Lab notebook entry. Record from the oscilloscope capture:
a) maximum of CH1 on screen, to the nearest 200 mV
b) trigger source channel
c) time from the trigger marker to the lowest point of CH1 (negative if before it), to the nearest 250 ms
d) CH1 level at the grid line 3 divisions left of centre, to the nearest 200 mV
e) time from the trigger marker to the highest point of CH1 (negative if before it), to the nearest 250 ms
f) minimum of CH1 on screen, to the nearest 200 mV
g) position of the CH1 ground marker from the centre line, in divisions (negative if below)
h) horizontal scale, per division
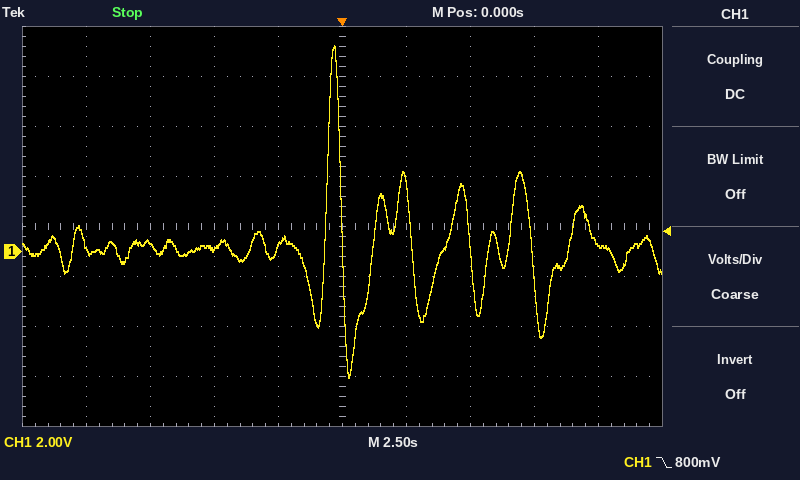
8.2 V
CH1
+250 ms
400 mV
-250 ms
-5.0 V
-0.5 div
2.5 s
